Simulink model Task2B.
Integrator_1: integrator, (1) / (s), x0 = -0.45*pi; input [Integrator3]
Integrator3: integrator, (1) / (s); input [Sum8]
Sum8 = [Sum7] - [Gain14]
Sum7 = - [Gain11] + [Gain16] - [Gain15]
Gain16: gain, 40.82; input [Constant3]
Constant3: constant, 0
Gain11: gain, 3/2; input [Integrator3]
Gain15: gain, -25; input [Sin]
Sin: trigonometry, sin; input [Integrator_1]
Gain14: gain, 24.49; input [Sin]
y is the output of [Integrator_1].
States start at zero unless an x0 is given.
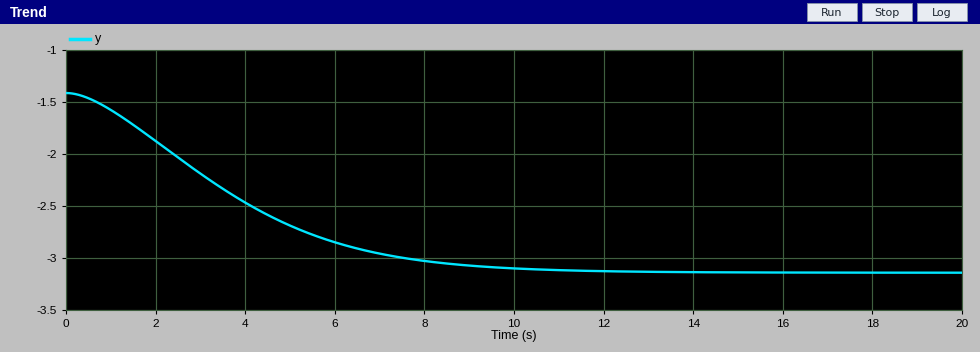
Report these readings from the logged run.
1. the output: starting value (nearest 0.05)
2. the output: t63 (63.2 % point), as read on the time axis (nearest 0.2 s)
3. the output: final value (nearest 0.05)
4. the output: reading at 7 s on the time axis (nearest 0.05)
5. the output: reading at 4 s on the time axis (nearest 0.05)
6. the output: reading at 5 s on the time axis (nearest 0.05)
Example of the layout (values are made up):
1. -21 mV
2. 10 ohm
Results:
1. -1.40
2. 4.2 s
3. -3.15
4. -2.95
5. -2.45
6. -2.70
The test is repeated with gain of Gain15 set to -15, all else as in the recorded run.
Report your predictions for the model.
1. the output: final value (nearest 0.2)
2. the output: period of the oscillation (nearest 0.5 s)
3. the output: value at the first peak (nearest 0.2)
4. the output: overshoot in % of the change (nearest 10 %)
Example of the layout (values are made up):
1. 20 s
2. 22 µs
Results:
1. 0.0
2. 2.0 s
3. 0.6
4. 40 %
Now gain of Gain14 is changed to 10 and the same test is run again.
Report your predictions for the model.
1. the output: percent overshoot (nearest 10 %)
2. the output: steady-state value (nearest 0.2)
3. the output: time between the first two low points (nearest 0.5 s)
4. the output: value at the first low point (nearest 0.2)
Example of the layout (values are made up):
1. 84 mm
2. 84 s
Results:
1. 50 %
2. -3.2
3. 1.5 s
4. -4.0
